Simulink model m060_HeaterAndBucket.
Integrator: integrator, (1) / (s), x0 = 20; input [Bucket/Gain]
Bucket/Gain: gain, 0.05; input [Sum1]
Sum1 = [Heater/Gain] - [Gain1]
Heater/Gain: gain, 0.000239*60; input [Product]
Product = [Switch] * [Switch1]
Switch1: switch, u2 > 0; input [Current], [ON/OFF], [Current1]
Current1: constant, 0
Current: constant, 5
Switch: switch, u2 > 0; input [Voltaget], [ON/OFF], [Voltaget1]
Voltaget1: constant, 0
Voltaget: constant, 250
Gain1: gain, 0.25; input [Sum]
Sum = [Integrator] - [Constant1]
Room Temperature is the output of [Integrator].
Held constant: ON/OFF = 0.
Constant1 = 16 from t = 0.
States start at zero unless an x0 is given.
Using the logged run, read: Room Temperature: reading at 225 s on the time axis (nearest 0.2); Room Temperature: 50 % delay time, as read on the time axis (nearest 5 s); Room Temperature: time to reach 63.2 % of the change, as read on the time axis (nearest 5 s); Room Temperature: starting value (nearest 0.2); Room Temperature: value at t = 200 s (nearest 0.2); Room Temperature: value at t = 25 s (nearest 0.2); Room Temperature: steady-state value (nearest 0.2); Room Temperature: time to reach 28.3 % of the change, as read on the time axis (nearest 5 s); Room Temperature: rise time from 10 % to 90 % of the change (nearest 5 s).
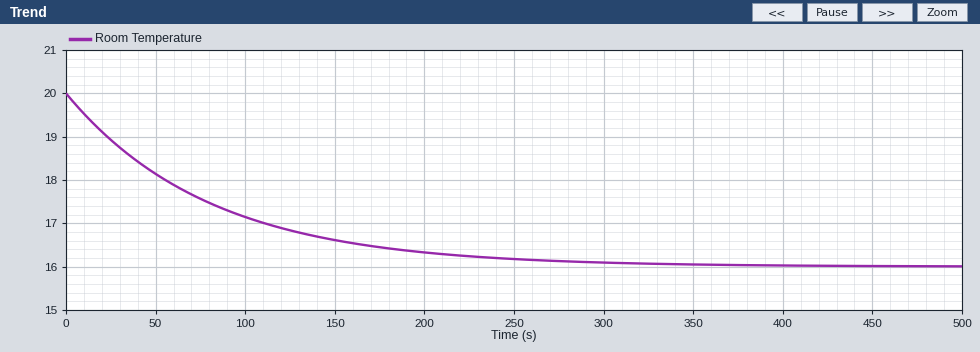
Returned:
16.2
55 s
80 s
20.0
16.4
19.0
16.0
25 s
175 s
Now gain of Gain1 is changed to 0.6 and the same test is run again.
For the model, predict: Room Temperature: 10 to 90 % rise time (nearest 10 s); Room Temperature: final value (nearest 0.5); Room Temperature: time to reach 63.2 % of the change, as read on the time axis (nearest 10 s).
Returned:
70 s
16.0
30 s
